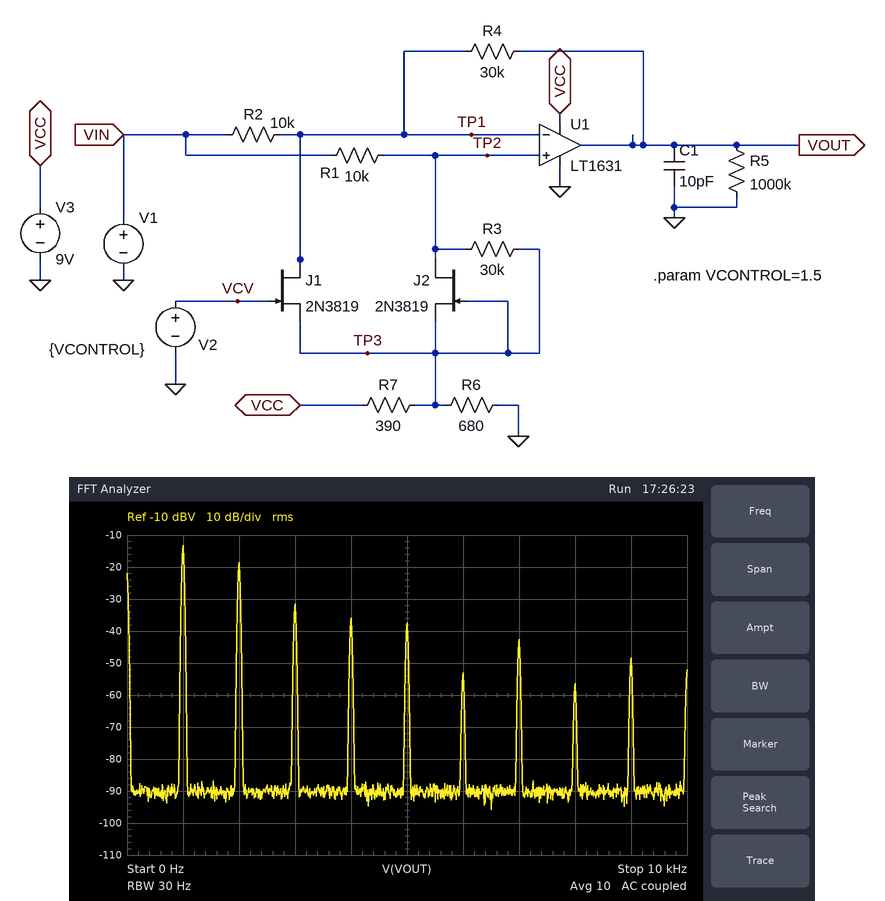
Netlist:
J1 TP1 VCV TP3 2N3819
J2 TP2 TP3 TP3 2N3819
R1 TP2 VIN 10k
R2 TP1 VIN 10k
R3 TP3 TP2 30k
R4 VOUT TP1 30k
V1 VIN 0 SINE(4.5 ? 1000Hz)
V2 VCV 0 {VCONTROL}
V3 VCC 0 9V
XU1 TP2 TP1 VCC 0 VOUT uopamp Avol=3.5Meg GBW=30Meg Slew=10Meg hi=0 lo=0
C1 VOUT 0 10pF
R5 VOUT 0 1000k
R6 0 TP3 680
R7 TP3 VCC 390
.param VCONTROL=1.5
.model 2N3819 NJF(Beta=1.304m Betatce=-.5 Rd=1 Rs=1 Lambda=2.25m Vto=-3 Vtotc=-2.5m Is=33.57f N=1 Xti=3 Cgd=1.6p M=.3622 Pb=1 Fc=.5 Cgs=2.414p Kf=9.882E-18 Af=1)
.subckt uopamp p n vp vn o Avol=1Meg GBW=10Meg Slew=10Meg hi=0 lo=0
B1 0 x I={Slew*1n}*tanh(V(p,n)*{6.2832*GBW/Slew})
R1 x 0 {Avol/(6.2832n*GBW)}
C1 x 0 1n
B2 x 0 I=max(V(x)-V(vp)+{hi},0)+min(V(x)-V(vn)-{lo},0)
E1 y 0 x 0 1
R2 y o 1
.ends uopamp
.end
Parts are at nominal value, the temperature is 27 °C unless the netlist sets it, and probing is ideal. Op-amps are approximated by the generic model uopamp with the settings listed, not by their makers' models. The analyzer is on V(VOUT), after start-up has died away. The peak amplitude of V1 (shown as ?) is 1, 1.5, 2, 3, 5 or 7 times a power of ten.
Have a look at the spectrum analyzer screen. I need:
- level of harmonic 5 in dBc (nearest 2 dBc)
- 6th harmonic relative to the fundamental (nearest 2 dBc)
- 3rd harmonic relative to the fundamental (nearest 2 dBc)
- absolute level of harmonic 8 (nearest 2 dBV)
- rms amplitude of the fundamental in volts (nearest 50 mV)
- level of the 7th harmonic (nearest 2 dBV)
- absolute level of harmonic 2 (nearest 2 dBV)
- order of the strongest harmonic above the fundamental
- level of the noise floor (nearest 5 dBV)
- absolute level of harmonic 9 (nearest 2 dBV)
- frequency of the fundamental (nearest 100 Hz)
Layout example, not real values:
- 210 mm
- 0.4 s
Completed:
- -24 dBc
- -40 dBc
- -18 dBc
- -56 dBV
- 200 mV
- -42 dBV
- -18 dBV
- 2
- -90 dBV
- -48 dBV
- 1.0 kHz
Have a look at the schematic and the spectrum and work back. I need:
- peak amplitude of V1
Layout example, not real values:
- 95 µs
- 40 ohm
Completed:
- 300 mV
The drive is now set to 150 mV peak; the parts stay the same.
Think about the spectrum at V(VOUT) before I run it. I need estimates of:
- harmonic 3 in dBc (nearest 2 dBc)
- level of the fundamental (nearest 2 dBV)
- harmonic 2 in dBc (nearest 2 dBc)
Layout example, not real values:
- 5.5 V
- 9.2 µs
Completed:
- -10 dBc
- -24 dBV
- -4 dBc
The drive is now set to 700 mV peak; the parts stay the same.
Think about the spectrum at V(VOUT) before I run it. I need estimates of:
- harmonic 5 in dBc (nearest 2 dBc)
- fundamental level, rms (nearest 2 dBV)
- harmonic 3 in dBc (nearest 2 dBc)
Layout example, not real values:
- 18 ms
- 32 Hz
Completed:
- -32 dBc
- -4 dBV
- -26 dBc
